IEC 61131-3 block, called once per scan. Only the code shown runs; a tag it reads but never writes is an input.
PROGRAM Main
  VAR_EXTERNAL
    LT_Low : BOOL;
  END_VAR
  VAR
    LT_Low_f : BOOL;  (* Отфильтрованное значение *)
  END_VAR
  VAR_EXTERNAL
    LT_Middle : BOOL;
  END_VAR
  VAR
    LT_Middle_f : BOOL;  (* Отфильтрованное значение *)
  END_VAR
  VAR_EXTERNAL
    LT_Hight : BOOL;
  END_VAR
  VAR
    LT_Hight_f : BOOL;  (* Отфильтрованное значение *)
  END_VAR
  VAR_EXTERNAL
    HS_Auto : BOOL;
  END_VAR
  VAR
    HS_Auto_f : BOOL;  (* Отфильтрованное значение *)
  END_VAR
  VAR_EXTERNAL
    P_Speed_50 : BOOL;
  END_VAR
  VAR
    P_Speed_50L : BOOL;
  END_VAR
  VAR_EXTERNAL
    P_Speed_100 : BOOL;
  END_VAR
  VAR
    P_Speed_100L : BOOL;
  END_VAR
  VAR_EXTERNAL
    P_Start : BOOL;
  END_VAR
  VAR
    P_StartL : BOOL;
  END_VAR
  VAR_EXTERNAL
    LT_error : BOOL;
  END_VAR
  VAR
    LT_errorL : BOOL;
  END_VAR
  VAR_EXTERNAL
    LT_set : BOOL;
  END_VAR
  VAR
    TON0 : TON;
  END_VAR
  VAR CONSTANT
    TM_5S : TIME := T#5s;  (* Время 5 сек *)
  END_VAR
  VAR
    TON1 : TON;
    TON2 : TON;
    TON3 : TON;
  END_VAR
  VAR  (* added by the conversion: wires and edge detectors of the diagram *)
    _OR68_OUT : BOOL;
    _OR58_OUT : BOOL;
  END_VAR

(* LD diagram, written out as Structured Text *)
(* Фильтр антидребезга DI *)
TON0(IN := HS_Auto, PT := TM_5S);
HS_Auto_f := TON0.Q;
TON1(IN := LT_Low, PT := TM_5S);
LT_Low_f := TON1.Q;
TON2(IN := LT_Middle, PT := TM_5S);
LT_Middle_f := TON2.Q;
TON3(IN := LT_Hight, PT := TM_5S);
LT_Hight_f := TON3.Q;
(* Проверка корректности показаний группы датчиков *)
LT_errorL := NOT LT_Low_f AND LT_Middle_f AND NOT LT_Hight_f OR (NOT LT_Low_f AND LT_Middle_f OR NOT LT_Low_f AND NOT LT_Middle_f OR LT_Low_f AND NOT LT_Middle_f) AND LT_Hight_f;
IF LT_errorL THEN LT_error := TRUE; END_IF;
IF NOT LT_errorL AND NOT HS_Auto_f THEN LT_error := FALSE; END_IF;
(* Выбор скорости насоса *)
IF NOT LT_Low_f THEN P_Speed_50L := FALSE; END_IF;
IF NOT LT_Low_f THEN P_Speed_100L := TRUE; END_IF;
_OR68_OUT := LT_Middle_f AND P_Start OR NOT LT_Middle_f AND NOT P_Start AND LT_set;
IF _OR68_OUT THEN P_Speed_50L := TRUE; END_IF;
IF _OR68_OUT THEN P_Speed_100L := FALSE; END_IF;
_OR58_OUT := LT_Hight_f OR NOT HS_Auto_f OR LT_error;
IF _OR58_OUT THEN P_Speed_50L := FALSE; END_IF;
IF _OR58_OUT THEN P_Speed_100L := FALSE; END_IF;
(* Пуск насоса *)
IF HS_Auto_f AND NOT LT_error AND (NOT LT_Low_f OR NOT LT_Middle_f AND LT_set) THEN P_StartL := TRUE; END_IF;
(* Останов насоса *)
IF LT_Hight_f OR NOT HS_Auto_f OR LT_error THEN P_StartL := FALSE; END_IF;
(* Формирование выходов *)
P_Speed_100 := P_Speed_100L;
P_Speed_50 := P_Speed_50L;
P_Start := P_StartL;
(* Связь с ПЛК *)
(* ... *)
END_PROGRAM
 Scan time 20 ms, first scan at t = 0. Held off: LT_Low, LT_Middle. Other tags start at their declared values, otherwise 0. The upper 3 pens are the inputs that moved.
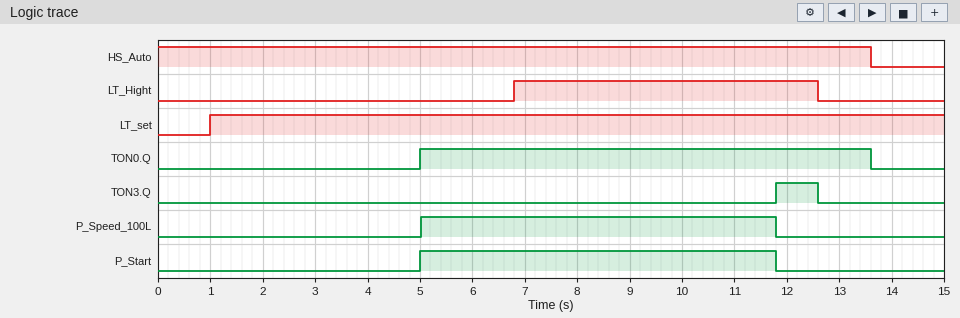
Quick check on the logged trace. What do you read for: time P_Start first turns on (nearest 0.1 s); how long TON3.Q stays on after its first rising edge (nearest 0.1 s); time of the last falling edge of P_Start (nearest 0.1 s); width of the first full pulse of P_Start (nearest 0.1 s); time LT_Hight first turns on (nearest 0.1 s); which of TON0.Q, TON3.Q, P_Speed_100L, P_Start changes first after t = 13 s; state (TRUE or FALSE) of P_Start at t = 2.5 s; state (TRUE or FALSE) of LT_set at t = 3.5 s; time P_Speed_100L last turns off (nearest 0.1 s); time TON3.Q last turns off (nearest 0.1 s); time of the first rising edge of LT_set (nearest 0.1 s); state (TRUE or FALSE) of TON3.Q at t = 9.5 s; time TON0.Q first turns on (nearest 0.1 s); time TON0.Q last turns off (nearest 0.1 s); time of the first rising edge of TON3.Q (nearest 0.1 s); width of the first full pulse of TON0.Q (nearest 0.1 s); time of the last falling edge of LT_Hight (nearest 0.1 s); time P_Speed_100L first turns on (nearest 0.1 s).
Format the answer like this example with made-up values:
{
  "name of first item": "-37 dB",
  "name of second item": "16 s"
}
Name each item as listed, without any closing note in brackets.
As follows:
{
  "time P_Start first turns on": "5.0 s",
  "how long TON3.Q stays on after its first rising edge": "0.8 s",
  "time of the last falling edge of P_Start": "11.8 s",
  "width of the first full pulse of P_Start": "6.8 s",
  "time LT_Hight first turns on": "6.8 s",
  "which of TON0.Q, TON3.Q, P_Speed_100L, P_Start changes first after t = 13 s": "TON0.Q",
  "state (TRUE or FALSE) of P_Start at t = 2.5 s": "FALSE",
  "state (TRUE or FALSE) of LT_set at t = 3.5 s": "TRUE",
  "time P_Speed_100L last turns off": "11.8 s",
  "time TON3.Q last turns off": "12.6 s",
  "time of the first rising edge of LT_set": "1.0 s",
  "state (TRUE or FALSE) of TON3.Q at t = 9.5 s": "FALSE",
  "time TON0.Q first turns on": "5.0 s",
  "time TON0.Q last turns off": "13.6 s",
  "time of the first rising edge of TON3.Q": "11.8 s",
  "width of the first full pulse of TON0.Q": "8.6 s",
  "time of the last falling edge of LT_Hight": "12.6 s",
  "time P_Speed_100L first turns on": "5.0 s"
}
